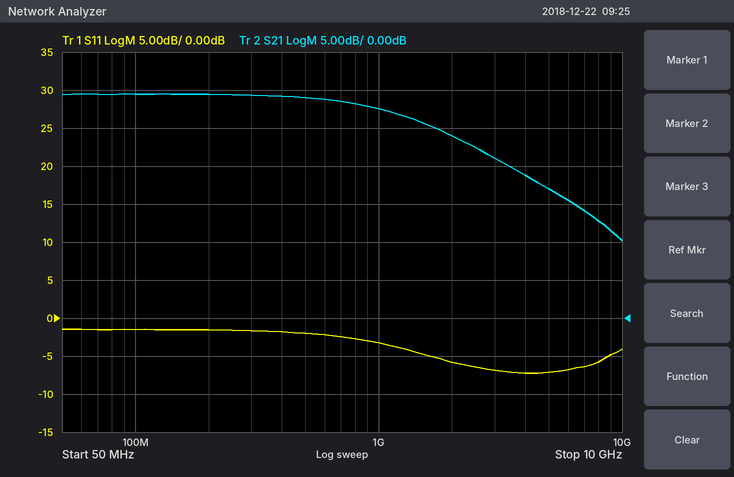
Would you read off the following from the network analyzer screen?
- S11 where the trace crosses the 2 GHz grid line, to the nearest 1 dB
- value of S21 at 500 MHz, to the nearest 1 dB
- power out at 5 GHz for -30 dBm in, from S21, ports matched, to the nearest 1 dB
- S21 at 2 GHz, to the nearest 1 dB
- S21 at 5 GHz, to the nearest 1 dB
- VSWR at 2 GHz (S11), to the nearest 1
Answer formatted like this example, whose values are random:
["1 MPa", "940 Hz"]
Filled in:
["-6 dB", "29 dB", "-13 dBm", "24 dB", "17 dB", "3"]
